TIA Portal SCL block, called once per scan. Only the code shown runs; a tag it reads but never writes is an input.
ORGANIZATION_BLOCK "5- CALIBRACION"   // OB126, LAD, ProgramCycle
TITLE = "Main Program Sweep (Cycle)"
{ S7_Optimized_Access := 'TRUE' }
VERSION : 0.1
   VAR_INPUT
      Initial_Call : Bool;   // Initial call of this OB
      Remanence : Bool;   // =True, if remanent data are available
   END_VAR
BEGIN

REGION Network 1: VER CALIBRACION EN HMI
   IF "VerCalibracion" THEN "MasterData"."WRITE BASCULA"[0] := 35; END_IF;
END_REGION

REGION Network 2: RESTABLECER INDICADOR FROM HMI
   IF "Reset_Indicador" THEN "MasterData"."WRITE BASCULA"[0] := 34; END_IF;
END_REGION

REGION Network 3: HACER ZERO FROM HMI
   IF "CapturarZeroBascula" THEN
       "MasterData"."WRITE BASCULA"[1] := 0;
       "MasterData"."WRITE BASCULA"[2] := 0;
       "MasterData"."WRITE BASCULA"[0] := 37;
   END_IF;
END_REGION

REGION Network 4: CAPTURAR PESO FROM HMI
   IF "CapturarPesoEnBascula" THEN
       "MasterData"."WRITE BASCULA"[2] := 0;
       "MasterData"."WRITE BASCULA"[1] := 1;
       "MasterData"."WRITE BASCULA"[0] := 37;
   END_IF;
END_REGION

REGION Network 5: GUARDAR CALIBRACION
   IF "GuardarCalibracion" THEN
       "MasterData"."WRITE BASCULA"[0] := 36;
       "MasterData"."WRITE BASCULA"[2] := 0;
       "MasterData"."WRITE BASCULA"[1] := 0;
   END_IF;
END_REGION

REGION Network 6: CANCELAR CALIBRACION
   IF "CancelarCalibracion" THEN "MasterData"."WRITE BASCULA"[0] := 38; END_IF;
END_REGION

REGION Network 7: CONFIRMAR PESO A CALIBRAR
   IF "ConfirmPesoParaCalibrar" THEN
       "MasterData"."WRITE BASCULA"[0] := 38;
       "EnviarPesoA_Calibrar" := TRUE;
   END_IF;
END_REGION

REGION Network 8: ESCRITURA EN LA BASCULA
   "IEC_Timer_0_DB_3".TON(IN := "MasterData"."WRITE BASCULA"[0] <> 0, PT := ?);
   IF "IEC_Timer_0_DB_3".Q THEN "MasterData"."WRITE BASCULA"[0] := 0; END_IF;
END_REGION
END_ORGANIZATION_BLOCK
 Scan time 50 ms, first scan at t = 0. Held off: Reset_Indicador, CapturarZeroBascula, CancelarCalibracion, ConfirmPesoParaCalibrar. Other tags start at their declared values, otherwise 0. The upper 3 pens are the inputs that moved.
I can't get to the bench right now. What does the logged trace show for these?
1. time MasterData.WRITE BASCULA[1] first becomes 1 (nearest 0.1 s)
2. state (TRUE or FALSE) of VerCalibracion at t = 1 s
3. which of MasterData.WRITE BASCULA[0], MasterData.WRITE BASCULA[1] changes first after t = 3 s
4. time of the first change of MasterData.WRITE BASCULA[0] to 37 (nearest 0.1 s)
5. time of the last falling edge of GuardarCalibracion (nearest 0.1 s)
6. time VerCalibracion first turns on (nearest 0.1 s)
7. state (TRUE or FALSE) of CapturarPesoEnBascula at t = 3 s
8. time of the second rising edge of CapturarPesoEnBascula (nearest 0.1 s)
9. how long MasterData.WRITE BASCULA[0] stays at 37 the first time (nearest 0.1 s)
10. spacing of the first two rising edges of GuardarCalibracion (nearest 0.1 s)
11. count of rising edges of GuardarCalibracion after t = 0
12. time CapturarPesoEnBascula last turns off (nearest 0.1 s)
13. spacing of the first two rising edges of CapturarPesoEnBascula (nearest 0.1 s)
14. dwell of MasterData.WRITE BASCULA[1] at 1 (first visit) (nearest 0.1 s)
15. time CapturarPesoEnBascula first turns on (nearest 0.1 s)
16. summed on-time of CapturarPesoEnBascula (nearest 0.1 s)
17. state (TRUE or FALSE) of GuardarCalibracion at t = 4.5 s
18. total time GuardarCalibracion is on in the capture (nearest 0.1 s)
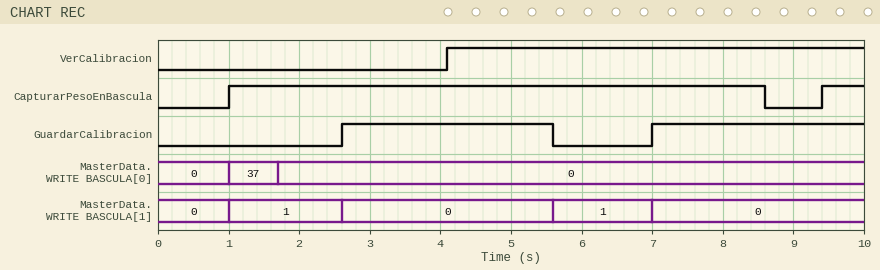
1.0 s
FALSE
MasterData.WRITE BASCULA[1]
1.0 s
5.6 s
4.1 s
TRUE
9.4 s
0.7 s
4.4 s
2
8.6 s
8.4 s
1.6 s
1.0 s
8.2 s
TRUE
6.0 s
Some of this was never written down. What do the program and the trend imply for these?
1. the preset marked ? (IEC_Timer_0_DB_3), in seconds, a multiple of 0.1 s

0.7 s
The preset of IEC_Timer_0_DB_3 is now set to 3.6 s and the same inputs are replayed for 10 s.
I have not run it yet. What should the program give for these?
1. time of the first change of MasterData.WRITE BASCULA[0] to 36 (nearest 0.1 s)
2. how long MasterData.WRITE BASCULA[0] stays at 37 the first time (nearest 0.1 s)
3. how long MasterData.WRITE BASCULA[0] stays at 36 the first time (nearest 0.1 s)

2.6 s
1.6 s
2.0 s
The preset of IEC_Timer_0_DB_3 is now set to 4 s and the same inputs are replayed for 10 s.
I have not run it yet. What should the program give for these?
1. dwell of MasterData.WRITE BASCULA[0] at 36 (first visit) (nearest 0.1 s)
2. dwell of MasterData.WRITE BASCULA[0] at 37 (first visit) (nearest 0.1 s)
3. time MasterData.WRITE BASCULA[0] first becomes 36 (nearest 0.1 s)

2.4 s
1.6 s
2.6 s
